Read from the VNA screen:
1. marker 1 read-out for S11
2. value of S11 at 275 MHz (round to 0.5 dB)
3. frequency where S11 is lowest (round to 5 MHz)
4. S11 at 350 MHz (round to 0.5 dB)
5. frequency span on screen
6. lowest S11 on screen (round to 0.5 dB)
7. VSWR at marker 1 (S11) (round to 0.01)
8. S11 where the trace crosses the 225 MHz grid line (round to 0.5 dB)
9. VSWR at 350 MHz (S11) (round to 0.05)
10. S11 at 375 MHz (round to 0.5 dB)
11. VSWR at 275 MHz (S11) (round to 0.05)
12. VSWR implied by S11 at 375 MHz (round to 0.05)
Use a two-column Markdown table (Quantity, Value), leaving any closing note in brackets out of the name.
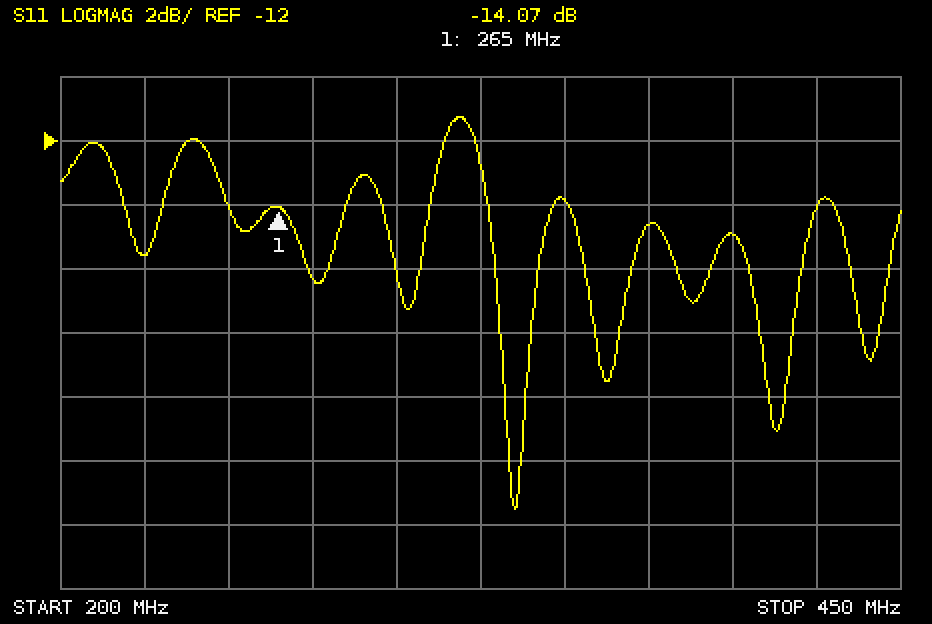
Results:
| Quantity | Value |
|---|---|
| marker 1 read-out for S11 | -14.07 dB |
| value of S11 at 275 MHz | -16.5 dB |
| frequency where S11 is lowest | 335 MHz |
| S11 at 350 MHz | -14.0 dB |
| frequency span on screen | 250 MHz |
| lowest S11 on screen | -23.5 dB |
| VSWR at marker 1 (S11) | 1.49 |
| S11 where the trace crosses the 225 MHz grid line | -15.5 dB |
| VSWR at 350 MHz (S11) | 1.50 |
| S11 at 375 MHz | -14.5 dB |
| VSWR at 275 MHz (S11) | 1.35 |
| VSWR implied by S11 at 375 MHz | 1.45 |
